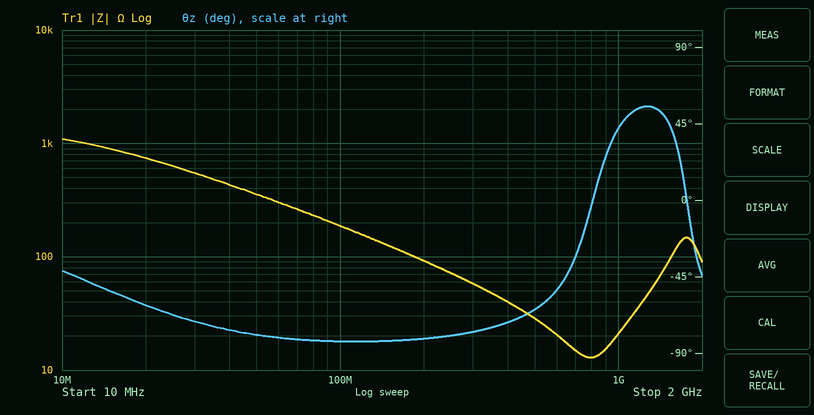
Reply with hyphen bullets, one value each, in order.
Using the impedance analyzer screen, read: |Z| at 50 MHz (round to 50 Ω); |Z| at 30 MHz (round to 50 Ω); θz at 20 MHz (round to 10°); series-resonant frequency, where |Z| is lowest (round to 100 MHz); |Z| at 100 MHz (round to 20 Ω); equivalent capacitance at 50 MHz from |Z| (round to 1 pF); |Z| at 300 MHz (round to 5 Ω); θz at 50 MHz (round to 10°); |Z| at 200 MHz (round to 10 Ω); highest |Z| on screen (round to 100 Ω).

- 350 Ω
- 550 Ω
- -60°
- 800 MHz
- 180 Ω
- 9 pF
- 60 Ω
- -80°
- 90 Ω
- 1.1 kΩ
